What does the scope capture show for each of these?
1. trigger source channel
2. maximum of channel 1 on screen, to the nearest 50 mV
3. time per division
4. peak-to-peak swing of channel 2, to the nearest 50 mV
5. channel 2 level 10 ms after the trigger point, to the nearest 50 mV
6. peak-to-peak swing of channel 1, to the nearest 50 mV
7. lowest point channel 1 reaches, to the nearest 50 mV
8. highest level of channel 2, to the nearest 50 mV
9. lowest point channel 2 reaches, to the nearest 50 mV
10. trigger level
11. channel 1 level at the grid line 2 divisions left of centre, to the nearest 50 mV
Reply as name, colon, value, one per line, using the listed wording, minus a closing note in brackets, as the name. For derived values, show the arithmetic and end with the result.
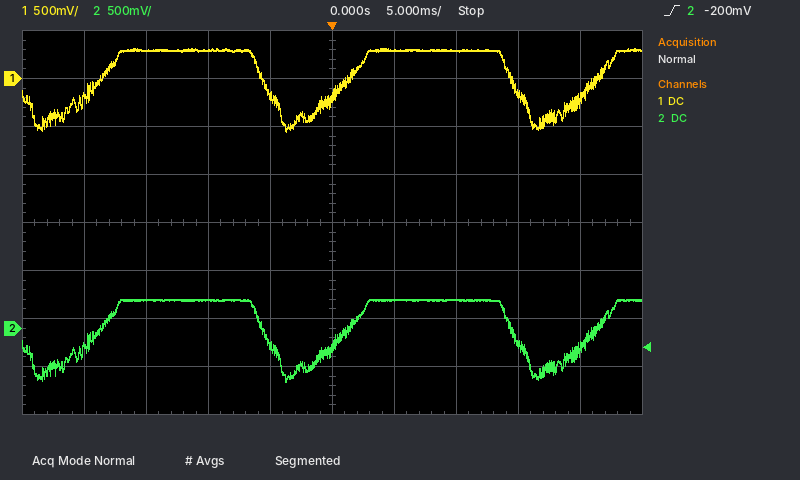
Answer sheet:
trigger source channel: channel 2
maximum of channel 1 on screen, to the nearest 50 mV: 300 mV
time per division: 5 ms
peak-to-peak swing of channel 2, to the nearest 50 mV: 300 mV − (-550 mV) = 850 mV
channel 2 level 10 ms after the trigger point, to the nearest 50 mV: 300 mV
peak-to-peak swing of channel 1, to the nearest 50 mV: 300 mV − (-550 mV) = 850 mV
lowest point channel 1 reaches, to the nearest 50 mV: -550 mV
highest level of channel 2, to the nearest 50 mV: 300 mV
lowest point channel 2 reaches, to the nearest 50 mV: -550 mV
trigger level: -200 mV
channel 1 level at the grid line 2 divisions left of centre, to the nearest 50 mV: 300 mV
